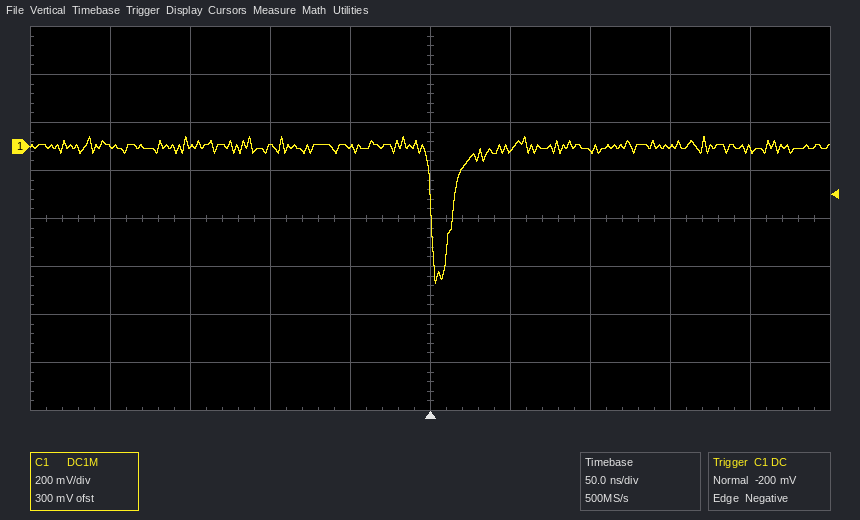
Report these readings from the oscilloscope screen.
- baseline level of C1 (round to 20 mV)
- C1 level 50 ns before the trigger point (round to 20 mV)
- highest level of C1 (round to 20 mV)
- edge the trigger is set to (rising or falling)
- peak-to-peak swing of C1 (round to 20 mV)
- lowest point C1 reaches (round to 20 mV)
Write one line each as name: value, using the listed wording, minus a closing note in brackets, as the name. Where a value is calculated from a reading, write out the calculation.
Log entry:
baseline level of C1: 0 mV
C1 level 50 ns before the trigger point: 0 mV
highest level of C1: 40 mV
edge the trigger is set to: falling
peak-to-peak swing of C1: 40 mV − (-580 mV) = 620 mV
lowest point C1 reaches: -580 mV
